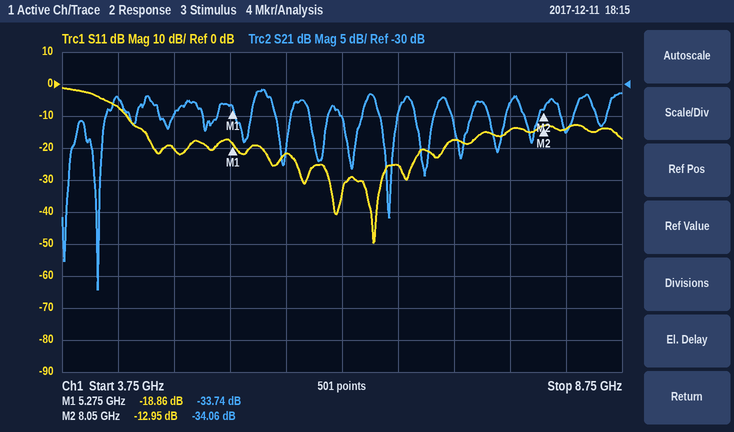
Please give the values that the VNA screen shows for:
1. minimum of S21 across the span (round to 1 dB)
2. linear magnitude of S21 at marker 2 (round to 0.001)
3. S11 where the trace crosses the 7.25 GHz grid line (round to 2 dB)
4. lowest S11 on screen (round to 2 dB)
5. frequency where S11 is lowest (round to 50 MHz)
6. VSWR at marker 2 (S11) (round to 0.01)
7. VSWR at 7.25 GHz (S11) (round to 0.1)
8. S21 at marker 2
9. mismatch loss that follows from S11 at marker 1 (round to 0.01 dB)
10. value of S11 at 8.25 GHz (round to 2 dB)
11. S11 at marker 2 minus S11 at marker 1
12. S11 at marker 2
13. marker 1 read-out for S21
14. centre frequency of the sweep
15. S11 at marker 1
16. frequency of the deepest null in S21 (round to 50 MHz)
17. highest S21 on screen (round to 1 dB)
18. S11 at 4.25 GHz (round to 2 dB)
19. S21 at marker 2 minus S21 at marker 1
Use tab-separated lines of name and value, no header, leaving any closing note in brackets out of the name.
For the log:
minimum of S21 across the span	-62 dB
linear magnitude of S21 at marker 2	0.020
S11 where the trace crosses the 7.25 GHz grid line	-18 dB
lowest S11 on screen	-50 dB
frequency where S11 is lowest	6.55 GHz
VSWR at marker 2 (S11)	1.58
VSWR at 7.25 GHz (S11)	1.3
S21 at marker 2	-34.06 dB
mismatch loss that follows from S11 at marker 1	0.06 dB
value of S11 at 8.25 GHz	-14 dB
S11 at marker 2 minus S11 at marker 1	5.91 dB
S11 at marker 2	-12.95 dB
marker 1 read-out for S21	-33.74 dB
centre frequency of the sweep	6.25 GHz
S11 at marker 1	-18.86 dB
frequency of the deepest null in S21	4.05 GHz
highest S21 on screen	-31 dB
S11 at 4.25 GHz	-8 dB
S21 at marker 2 minus S21 at marker 1	-0.32 dB
